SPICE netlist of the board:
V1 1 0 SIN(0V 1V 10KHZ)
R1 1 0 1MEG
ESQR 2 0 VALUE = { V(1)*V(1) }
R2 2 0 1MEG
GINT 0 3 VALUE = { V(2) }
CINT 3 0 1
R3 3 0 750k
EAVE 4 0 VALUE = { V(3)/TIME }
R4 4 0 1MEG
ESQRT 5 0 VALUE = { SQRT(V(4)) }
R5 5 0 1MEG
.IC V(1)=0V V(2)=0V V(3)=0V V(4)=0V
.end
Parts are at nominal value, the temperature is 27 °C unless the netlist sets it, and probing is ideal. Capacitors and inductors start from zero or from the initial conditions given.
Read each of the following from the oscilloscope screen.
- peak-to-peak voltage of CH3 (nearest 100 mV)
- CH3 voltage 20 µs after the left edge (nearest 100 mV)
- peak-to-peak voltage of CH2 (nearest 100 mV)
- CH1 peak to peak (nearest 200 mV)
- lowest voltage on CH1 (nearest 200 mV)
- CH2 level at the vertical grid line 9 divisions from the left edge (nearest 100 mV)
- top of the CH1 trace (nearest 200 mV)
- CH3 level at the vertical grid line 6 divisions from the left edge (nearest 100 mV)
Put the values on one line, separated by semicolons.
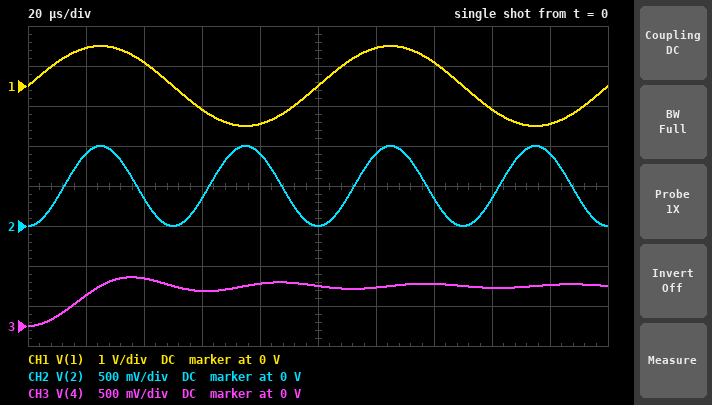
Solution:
600 mV; 400 mV; 1.0 V; 2.0 V; -1.0 V; 900 mV; 1.0 V; 500 mV
